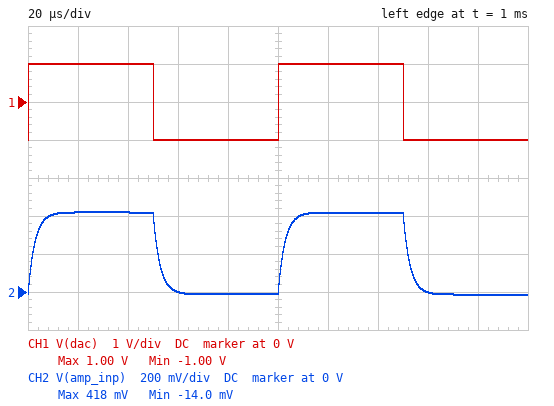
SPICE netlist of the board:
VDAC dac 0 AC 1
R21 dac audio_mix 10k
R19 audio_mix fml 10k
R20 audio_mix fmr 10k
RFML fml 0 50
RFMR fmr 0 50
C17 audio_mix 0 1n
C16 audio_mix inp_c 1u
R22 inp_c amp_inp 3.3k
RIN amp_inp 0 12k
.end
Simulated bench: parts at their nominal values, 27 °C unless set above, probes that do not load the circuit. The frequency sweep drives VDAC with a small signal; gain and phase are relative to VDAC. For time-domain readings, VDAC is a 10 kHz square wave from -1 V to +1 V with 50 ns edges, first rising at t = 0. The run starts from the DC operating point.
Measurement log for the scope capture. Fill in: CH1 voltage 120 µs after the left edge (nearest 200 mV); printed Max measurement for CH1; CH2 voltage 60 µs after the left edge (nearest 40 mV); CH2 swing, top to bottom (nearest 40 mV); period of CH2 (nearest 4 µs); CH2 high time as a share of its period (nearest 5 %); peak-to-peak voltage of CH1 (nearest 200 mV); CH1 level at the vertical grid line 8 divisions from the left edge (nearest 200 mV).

1.0 V
1.00 V
0 V
440 mV
100 µs
50 %
2.0 V
-1.0 V
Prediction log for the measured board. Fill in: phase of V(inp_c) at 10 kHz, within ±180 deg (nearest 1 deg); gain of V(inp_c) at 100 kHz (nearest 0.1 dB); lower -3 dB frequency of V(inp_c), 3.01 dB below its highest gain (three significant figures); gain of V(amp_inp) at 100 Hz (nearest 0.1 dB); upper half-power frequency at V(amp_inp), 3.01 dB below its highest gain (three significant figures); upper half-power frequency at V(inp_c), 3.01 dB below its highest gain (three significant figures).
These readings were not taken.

-10 deg
-17.2 dB
8.53 Hz
-13.4 dB
58.0 kHz
58.0 kHz
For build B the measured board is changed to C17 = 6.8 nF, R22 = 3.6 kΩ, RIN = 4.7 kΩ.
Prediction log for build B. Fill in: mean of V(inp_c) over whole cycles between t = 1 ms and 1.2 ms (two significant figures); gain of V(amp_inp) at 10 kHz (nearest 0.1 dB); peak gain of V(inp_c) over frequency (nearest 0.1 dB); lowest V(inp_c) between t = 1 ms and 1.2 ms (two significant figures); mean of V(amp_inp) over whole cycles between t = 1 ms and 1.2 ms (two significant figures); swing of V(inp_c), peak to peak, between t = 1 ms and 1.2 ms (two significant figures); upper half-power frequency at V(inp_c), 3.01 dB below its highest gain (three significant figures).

220 mV
-20.5 dB
-12.5 dB
-2.4 mV
120 mV
440 mV
9.85 kHz
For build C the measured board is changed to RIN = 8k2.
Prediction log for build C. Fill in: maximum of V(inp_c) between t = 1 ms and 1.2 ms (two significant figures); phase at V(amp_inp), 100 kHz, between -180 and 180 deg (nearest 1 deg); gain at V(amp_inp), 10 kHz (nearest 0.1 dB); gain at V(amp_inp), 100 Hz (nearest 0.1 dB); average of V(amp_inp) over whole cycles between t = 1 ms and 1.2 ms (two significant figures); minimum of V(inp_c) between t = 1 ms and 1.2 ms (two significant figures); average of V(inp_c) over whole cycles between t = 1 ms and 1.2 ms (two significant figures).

500 mV
-58 deg
-14.8 dB
-14.7 dB
170 mV
-20 mV
240 mV
